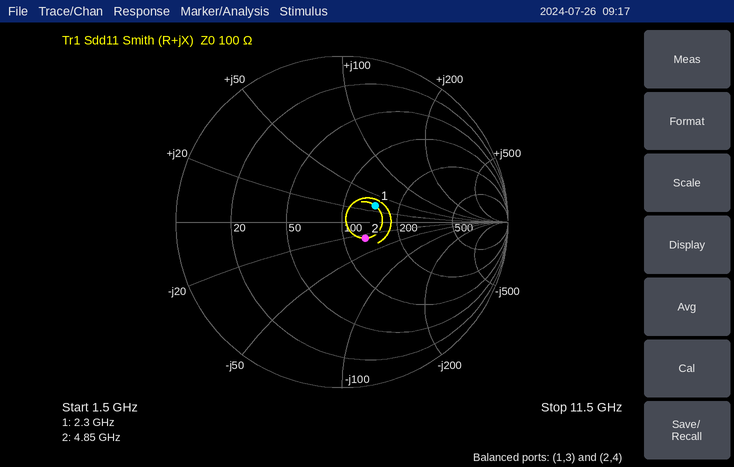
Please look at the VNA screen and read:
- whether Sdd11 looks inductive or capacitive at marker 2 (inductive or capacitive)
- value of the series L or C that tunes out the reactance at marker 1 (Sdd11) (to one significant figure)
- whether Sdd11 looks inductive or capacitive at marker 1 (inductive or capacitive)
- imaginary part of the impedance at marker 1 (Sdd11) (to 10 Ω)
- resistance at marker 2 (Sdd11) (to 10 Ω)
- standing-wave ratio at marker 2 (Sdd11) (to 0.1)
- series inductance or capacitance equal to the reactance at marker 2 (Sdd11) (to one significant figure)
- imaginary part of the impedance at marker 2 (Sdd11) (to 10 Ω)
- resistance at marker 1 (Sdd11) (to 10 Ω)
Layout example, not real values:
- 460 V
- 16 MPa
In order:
- capacitive
- 2 pF
- inductive
- +30 Ω
- 130 Ω
- 1.4
- 1 pF
- -30 Ω
- 150 Ω
